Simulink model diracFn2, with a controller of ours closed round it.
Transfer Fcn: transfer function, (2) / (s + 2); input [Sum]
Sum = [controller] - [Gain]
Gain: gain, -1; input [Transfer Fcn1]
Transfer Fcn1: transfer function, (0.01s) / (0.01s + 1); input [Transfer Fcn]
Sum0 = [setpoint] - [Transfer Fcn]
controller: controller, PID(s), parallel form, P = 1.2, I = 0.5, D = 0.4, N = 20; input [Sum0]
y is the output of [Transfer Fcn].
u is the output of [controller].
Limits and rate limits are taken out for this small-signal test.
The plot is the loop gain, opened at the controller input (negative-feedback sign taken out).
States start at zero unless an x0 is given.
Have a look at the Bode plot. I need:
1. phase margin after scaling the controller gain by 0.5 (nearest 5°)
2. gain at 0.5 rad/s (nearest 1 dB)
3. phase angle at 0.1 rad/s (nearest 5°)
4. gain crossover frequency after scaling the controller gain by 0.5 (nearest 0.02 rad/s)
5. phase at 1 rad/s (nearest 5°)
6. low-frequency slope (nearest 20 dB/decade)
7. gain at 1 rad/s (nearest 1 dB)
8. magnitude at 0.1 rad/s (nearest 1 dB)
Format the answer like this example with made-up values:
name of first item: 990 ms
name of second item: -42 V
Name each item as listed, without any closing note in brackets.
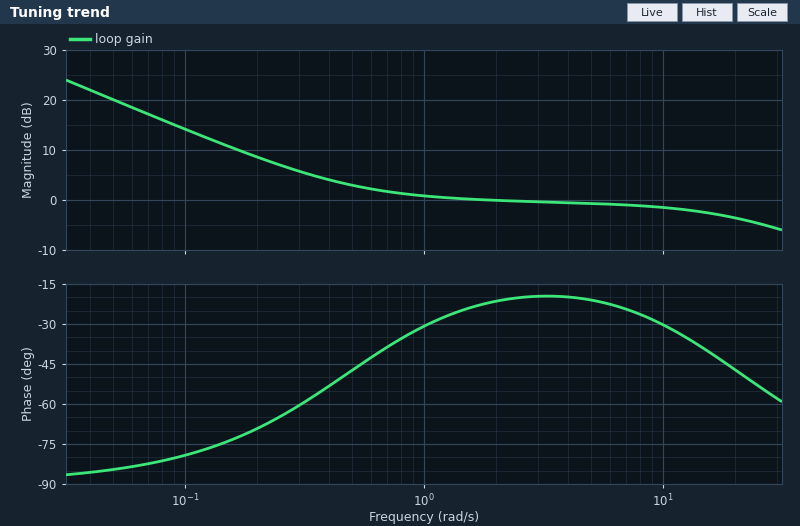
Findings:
phase margin after scaling the controller gain by 0.5: 120°
gain at 0.5 rad/s: 3 dB
phase angle at 0.1 rad/s: -80°
gain crossover frequency after scaling the controller gain by 0.5: 0.28 rad/s
phase at 1 rad/s: -30°
low-frequency slope: -20 dB/decade
gain at 1 rad/s: 1 dB
magnitude at 0.1 rad/s: 14 dB
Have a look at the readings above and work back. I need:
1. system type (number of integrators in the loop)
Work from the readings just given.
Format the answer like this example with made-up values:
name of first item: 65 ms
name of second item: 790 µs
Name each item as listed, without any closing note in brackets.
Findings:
system type: 1
